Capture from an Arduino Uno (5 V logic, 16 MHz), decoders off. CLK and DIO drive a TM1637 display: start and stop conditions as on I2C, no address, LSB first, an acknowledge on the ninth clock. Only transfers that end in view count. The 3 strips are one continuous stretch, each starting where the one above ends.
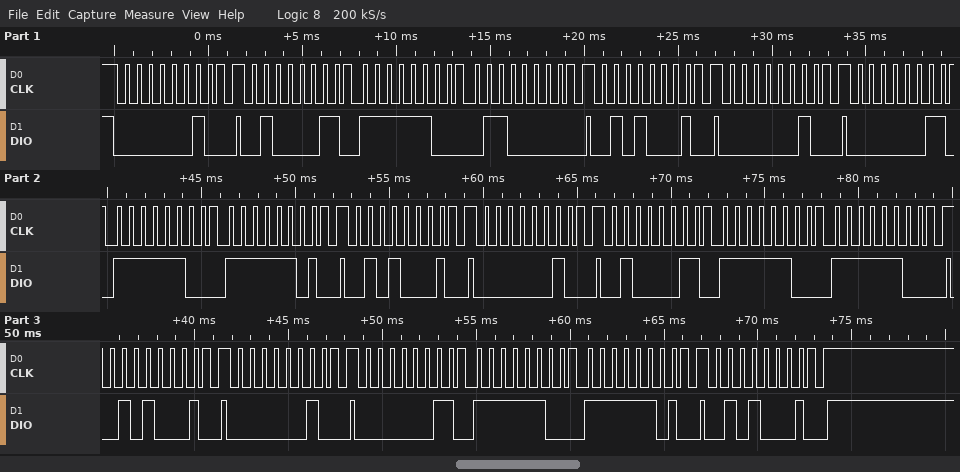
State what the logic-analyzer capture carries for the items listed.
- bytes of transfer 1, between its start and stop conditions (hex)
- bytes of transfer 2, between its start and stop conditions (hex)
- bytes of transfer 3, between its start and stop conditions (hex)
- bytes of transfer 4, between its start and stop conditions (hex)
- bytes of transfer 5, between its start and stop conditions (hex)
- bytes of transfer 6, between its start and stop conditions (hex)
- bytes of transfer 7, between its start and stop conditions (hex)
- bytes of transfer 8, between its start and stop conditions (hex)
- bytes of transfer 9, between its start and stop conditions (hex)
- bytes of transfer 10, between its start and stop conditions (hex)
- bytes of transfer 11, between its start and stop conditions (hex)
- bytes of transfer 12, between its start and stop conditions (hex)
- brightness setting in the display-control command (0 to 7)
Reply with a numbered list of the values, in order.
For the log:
1. 40
2. C2 3F 06
3. 8A
4. 40
5. C0 3F BF
6. 8A
7. 40
8. C2 3F 3F
9. 8A
10. 40
11. C0 3F BF
12. 8A
13. 2
